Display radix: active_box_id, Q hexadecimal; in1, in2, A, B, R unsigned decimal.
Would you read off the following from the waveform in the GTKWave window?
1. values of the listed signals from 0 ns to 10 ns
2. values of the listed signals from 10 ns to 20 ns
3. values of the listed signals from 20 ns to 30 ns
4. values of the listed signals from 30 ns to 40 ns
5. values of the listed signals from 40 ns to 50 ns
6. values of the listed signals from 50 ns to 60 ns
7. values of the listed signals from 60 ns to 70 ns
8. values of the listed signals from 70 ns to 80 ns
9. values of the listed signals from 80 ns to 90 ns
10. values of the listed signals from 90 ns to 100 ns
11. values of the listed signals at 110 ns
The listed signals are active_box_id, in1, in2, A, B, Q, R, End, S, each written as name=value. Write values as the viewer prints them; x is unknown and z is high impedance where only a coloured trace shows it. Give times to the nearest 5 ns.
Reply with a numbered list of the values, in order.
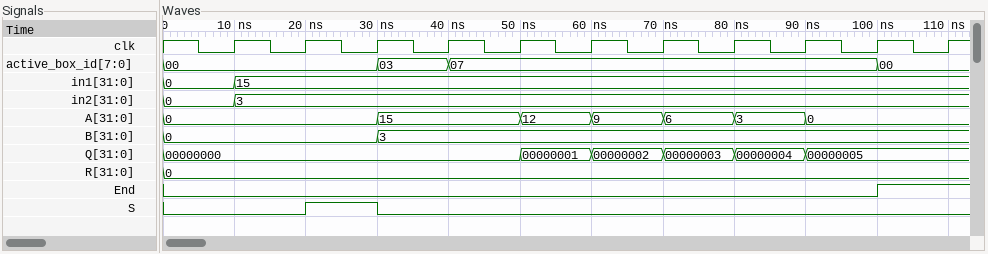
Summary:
1. active_box_id=00, in1=0, in2=0, A=0, B=0, Q=00000000, R=0, End=0, S=0
2. active_box_id=00, in1=15, in2=3, A=0, B=0, Q=00000000, R=0, End=0, S=0
3. active_box_id=00, in1=15, in2=3, A=0, B=0, Q=00000000, R=0, End=0, S=1
4. active_box_id=03, in1=15, in2=3, A=15, B=3, Q=00000000, R=0, End=0, S=0
5. active_box_id=07, in1=15, in2=3, A=15, B=3, Q=00000000, R=0, End=0, S=0
6. active_box_id=07, in1=15, in2=3, A=12, B=3, Q=00000001, R=0, End=0, S=0
7. active_box_id=07, in1=15, in2=3, A=9, B=3, Q=00000002, R=0, End=0, S=0
8. active_box_id=07, in1=15, in2=3, A=6, B=3, Q=00000003, R=0, End=0, S=0
9. active_box_id=07, in1=15, in2=3, A=3, B=3, Q=00000004, R=0, End=0, S=0
10. active_box_id=07, in1=15, in2=3, A=0, B=3, Q=00000005, R=0, End=0, S=0
11. active_box_id=00, in1=15, in2=3, A=0, B=3, Q=00000005, R=0, End=1, S=0
